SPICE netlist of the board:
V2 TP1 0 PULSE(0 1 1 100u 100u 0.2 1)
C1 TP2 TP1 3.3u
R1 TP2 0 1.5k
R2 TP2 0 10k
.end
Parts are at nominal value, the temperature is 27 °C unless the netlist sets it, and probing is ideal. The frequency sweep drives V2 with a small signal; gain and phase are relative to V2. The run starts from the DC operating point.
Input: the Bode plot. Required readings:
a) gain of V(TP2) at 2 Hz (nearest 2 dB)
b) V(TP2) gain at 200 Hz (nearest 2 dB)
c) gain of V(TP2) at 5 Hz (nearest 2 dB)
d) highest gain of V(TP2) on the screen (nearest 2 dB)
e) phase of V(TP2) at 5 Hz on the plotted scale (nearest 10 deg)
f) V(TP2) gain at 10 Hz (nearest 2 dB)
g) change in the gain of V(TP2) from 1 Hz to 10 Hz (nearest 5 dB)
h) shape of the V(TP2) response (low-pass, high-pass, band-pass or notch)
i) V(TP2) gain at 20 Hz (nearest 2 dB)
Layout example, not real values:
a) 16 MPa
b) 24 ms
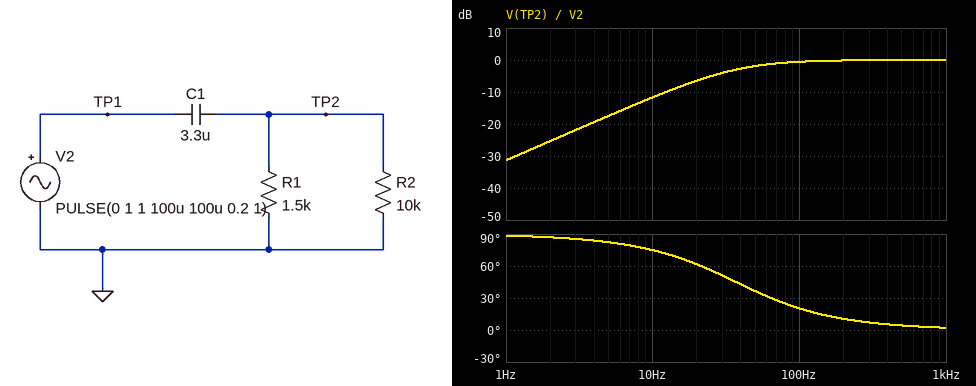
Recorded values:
a) -26 dB
b) 0 dB
c) -18 dB
d) 0 dB
e) 80 deg
f) -12 dB
g) 20 dB
h) high-pass
i) -6 dB
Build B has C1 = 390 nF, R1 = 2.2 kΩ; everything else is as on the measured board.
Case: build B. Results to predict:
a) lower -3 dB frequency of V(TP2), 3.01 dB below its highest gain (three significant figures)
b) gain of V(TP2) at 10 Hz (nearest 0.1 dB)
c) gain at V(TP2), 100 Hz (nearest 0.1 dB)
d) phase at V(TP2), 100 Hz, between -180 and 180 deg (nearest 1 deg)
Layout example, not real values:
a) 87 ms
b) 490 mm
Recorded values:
a) 226 Hz
b) -27.1 dB
c) -7.9 dB
d) 66 deg
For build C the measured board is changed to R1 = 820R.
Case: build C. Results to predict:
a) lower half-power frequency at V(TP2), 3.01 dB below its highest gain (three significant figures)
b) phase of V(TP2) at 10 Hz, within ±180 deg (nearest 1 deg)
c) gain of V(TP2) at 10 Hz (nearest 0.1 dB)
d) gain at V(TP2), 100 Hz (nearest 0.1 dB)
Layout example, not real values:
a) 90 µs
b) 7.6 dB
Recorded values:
a) 63.6 Hz
b) 81 deg
c) -16.2 dB
d) -1.5 dB
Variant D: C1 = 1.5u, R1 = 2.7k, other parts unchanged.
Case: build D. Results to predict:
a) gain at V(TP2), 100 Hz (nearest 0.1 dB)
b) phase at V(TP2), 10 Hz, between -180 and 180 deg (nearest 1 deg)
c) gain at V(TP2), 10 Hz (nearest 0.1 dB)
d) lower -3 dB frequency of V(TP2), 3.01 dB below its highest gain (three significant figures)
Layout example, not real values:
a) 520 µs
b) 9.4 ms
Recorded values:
a) -1.0 dB
b) 79 deg
c) -14.1 dB
d) 49.9 Hz
